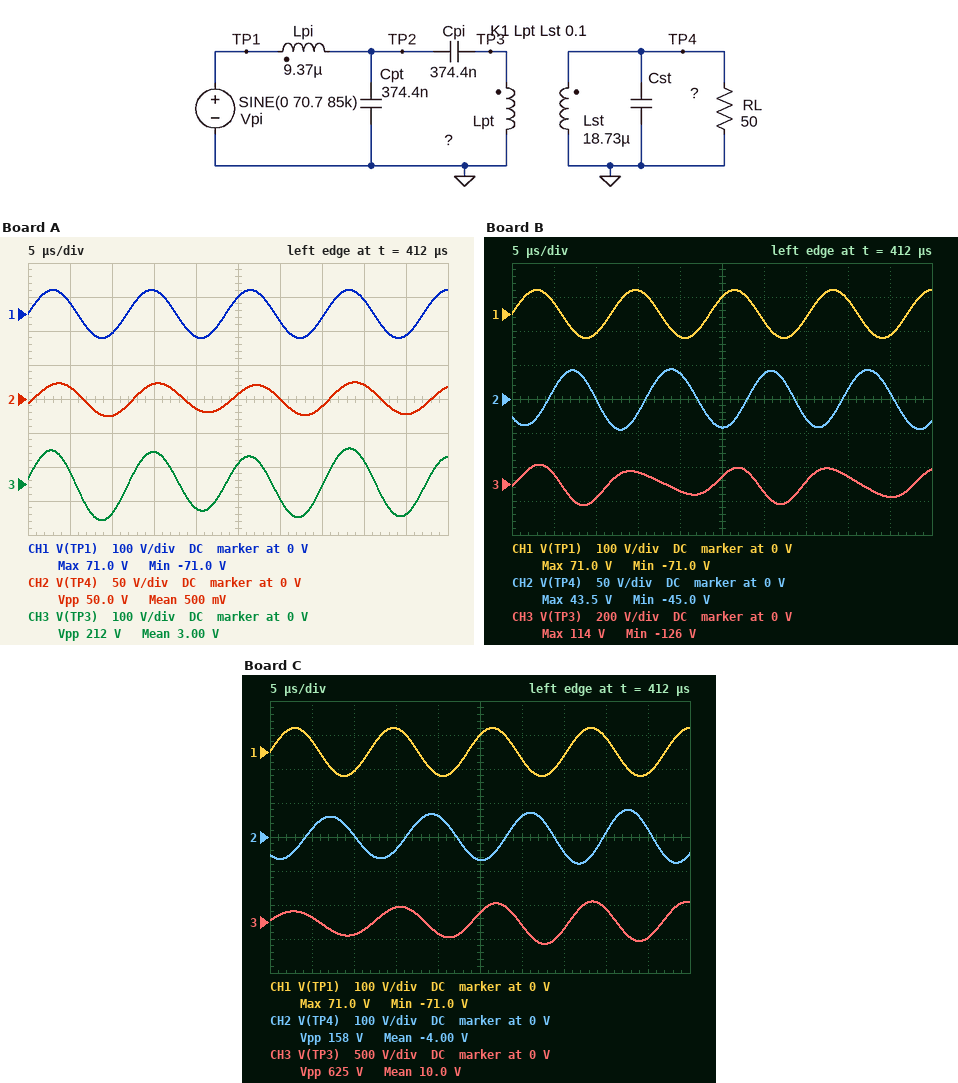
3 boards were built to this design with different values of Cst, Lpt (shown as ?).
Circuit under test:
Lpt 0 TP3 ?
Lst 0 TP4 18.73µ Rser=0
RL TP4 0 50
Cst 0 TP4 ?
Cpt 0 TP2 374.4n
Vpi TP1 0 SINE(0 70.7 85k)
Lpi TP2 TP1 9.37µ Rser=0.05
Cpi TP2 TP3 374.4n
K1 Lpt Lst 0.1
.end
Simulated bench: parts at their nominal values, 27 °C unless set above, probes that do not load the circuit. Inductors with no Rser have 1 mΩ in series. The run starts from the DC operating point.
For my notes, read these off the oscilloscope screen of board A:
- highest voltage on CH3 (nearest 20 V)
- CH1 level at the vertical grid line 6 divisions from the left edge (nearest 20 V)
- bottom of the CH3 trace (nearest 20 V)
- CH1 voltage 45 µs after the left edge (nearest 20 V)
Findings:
100 V
-20 V
-100 V
-60 V
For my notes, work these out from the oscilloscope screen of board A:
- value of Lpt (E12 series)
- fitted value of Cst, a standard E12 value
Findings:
12 µH
100 nF
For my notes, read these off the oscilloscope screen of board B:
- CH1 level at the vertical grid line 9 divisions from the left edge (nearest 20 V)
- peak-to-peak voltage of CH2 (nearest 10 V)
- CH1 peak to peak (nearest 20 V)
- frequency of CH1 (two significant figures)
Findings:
-60 V
90 V
140 V
85 kHz
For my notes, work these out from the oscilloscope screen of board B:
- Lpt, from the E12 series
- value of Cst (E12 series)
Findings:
12 µH
220 nF
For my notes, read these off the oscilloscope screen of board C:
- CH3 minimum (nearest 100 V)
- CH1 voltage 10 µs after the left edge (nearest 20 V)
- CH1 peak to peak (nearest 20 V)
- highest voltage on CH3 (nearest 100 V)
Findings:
-300 V
-60 V
140 V
300 V
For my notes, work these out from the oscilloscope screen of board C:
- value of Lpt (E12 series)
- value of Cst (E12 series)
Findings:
33 µH
220 nF
